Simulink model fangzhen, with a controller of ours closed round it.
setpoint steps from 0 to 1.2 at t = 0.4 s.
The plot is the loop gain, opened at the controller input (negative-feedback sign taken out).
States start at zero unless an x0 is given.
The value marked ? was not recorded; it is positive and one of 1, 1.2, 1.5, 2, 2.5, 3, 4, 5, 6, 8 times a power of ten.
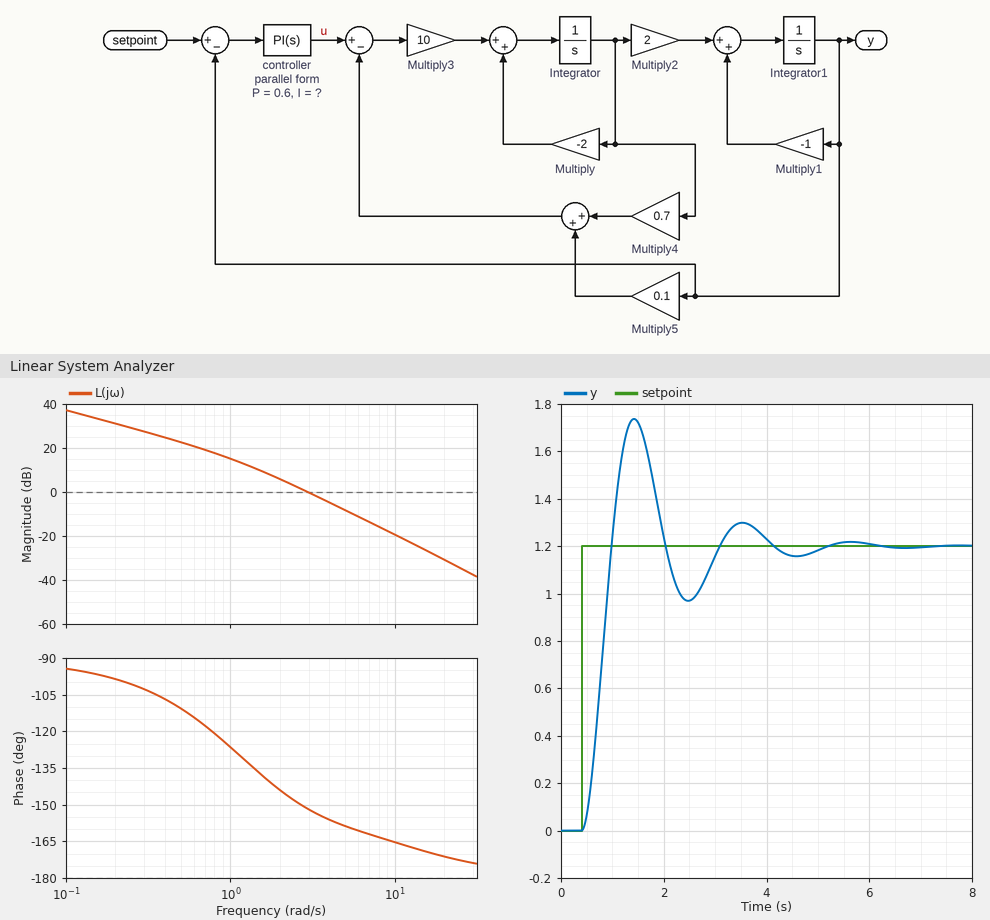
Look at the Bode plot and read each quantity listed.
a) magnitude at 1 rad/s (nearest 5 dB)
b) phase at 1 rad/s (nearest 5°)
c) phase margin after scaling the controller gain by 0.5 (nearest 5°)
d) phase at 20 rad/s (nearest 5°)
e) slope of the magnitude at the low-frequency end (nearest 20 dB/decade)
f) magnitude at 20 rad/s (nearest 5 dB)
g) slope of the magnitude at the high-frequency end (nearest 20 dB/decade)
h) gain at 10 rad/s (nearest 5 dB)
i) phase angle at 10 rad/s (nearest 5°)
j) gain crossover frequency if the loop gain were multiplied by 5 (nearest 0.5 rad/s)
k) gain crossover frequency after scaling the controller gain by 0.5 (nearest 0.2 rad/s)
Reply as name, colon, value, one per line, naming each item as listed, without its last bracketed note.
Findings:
magnitude at 1 rad/s: 15 dB
phase at 1 rad/s: -125°
phase margin after scaling the controller gain by 0.5: 35°
phase at 20 rad/s: -170°
slope of the magnitude at the low-frequency end: -20 dB/decade
magnitude at 20 rad/s: -30 dB
slope of the magnitude at the high-frequency end: -40 dB/decade
gain at 10 rad/s: -20 dB
phase angle at 10 rad/s: -165°
gain crossover frequency if the loop gain were multiplied by 5: 7.0 rad/s
gain crossover frequency after scaling the controller gain by 0.5: 2.0 rad/s
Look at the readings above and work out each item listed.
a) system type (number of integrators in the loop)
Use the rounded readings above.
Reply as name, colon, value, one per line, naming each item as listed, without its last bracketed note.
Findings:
system type: 1
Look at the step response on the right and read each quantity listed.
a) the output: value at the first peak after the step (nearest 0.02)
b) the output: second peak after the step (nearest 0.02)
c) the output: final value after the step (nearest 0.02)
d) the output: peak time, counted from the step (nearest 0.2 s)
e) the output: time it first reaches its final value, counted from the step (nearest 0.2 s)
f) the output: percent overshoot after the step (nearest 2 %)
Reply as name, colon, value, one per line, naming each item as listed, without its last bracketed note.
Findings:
the output: value at the first peak after the step: 1.74
the output: second peak after the step: 1.30
the output: final value after the step: 1.20
the output: peak time, counted from the step: 1.0 s
the output: time it first reaches its final value, counted from the step: 0.6 s
the output: percent overshoot after the step: 44 %
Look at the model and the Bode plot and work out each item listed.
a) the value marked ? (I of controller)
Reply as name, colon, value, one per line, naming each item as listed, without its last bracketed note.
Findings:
the value marked ?: 4
